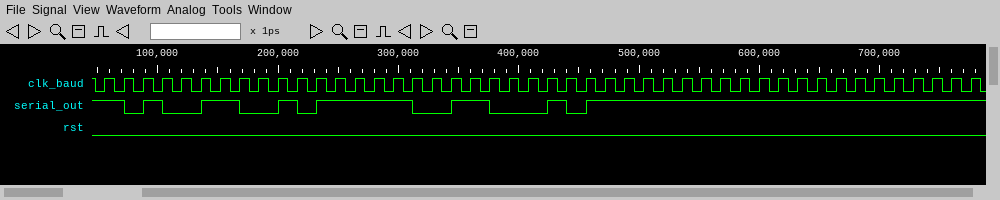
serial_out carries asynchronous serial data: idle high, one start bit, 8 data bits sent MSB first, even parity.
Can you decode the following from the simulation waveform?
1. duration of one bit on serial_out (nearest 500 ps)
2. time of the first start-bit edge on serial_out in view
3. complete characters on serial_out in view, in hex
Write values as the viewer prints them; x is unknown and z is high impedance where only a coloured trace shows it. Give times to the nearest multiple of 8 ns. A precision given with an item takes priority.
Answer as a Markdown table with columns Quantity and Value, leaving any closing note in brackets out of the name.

| Quantity | Value |
|---|---|
| duration of one bit on serial_out | 16000 ps |
| time of the first start-bit edge on serial_out in view | 72 ns |
| complete characters on serial_out in view, in hex | 99, 62 |
